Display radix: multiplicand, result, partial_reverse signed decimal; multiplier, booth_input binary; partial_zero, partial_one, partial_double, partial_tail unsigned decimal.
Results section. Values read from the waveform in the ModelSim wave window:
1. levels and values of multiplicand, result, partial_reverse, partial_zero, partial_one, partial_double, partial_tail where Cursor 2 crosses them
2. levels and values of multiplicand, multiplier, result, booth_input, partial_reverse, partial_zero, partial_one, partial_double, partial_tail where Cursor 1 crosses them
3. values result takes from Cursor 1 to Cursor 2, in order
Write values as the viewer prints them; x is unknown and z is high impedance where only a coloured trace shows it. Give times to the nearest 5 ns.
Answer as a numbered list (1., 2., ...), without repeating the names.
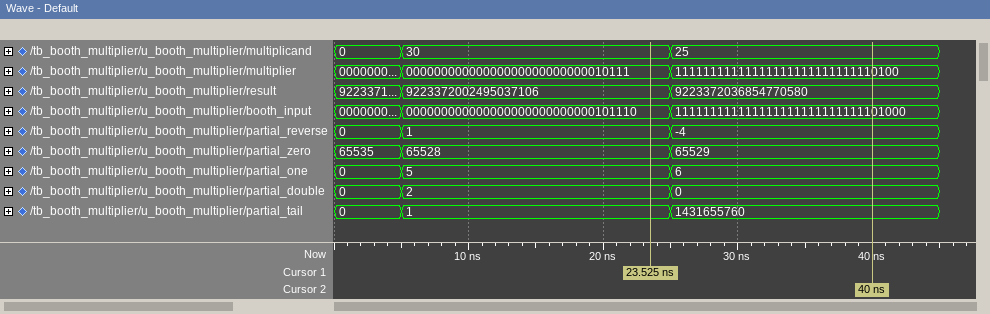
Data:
1. multiplicand=25, result=9223372036854770580, partial_reverse=-4, partial_zero=65529, partial_one=6, partial_double=0, partial_tail=1431655760
2. multiplicand=30, multiplier=00000000000000000000000000010111, result=9223372002495037106, booth_input=000000000000000000000000000101110, partial_reverse=1, partial_zero=65528, partial_one=5, partial_double=2, partial_tail=1
3. 9223372002495037106, 9223372036854770580
